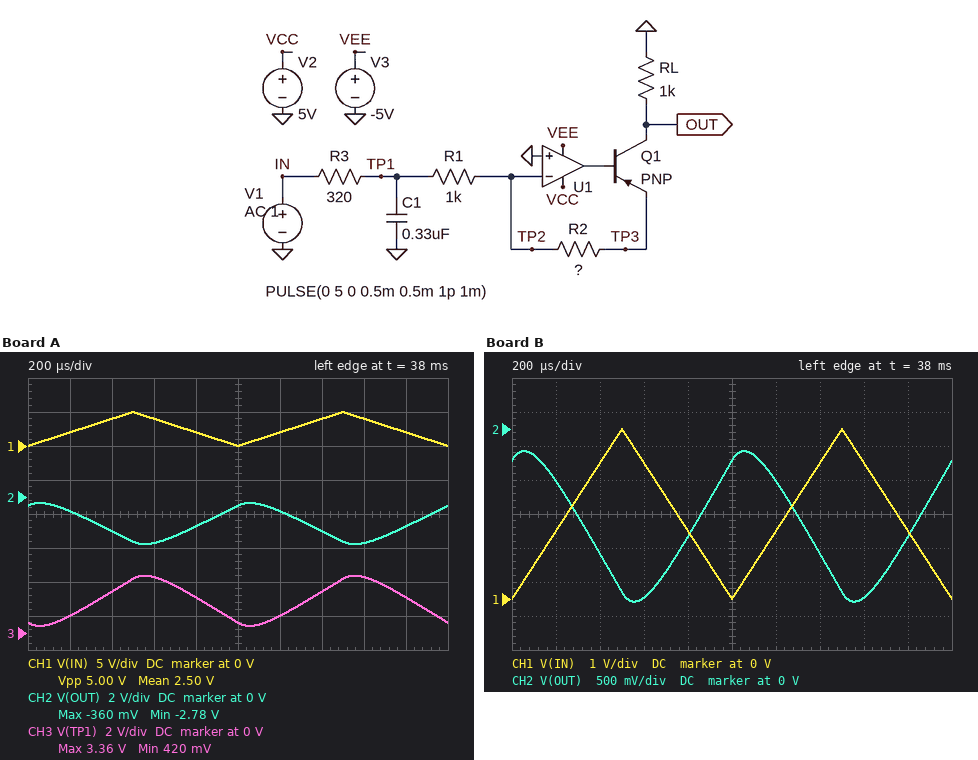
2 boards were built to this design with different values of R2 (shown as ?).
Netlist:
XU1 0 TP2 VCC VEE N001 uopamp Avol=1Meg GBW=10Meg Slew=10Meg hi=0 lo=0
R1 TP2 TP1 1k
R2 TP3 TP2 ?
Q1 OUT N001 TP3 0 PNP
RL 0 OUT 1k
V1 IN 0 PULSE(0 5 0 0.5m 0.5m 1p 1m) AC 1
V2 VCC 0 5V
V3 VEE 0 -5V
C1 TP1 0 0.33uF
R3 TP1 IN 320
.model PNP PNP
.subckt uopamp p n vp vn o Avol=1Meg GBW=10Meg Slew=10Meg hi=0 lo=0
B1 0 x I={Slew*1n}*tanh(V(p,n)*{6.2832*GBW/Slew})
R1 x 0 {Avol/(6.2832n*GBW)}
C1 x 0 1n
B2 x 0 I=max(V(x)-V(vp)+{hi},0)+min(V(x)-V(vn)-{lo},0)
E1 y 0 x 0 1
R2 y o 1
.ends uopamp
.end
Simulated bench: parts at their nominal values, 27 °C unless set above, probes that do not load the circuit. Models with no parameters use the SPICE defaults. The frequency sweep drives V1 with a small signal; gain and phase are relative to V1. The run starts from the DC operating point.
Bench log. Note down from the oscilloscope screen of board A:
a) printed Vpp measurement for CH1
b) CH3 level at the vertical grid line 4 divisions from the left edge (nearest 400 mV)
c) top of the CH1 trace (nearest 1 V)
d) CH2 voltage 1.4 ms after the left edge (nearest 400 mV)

5.00 V
2.0 V
5 V
-2.0 V
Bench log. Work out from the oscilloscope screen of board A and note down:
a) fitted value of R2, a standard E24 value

820 Ω
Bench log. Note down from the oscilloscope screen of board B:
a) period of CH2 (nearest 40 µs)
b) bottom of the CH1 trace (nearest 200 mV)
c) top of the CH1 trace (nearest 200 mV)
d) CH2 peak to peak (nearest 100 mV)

1.00 ms
0 V
5.0 V
2.2 V
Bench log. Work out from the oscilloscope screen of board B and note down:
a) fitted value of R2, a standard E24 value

750 Ω
